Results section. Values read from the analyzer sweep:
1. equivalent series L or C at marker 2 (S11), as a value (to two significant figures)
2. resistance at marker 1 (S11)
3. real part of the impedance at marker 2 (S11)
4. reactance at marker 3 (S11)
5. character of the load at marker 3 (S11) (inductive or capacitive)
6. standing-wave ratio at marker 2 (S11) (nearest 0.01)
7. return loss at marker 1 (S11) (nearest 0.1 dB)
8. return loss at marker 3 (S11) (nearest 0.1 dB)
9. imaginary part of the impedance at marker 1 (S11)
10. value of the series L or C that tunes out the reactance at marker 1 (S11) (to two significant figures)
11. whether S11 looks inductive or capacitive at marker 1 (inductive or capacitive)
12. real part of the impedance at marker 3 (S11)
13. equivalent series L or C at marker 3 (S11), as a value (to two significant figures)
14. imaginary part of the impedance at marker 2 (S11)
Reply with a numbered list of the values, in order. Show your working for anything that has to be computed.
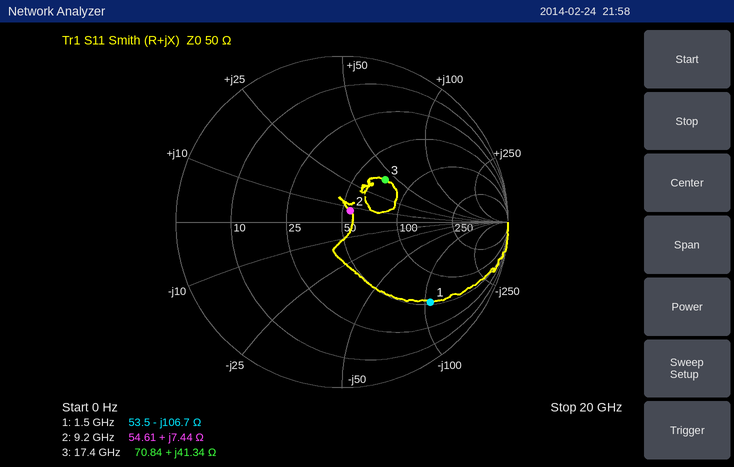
1. L = 7.44 Ω/(2π × 9.2 GHz) ≈ 129 pH, so 130 pH to two significant figures
2. 53.5 Ω
3. 54.61 Ω
4. +41.34 Ω
5. inductive
6. 1.18
7. 2.9 dB
8. 8.8 dB
9. -106.7 Ω
10. L = 106.7 Ω/(2π × 1.5 GHz) ≈ 11 nH
11. capacitive
12. 70.84 Ω
13. L = 41.34 Ω/(2π × 17.4 GHz) ≈ 378 pH, so 380 pH to two significant figures
14. +7.44 Ω
